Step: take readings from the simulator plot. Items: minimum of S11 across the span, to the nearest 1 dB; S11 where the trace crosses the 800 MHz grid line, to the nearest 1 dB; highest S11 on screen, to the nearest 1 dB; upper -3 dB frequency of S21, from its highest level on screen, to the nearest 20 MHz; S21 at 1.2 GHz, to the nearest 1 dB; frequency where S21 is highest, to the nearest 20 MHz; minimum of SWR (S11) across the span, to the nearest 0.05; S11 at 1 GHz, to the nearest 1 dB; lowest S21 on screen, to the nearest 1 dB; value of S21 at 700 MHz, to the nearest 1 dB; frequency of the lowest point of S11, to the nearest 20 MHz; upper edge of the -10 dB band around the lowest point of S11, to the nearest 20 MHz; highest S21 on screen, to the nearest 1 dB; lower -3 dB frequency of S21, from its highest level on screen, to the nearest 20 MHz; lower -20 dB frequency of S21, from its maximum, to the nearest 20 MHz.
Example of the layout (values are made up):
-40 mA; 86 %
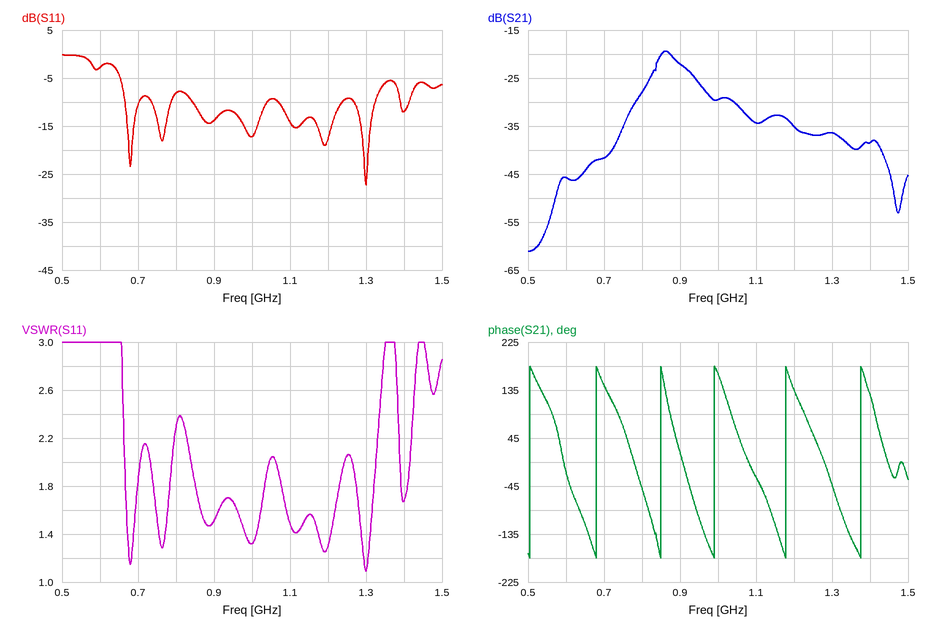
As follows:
-27 dB; -8 dB; 0 dB; 900 MHz; -35 dB; 860 MHz; 1.10; -17 dB; -61 dB; -42 dB; 1.30 GHz; 1.32 GHz; -19 dB; 840 MHz; 720 MHz
